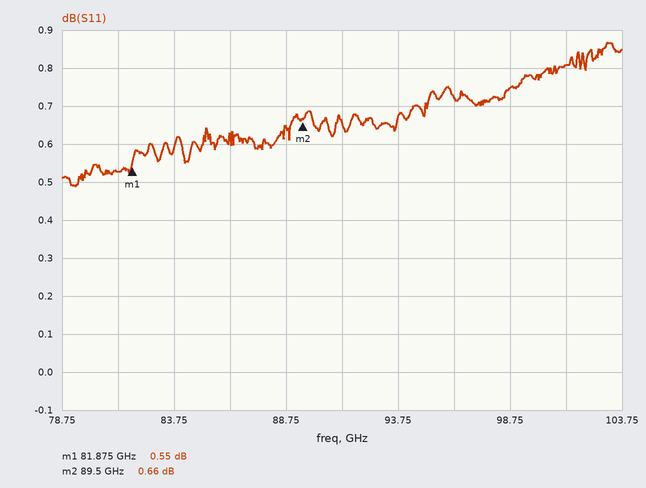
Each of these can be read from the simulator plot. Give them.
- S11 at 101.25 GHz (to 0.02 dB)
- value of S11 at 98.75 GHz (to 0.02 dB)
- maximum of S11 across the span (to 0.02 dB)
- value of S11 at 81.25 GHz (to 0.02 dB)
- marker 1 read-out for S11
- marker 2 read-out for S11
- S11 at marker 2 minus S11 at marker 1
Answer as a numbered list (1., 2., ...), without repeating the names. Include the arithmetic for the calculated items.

1. 0.80 dB
2. 0.74 dB
3. 0.86 dB
4. 0.52 dB
5. 0.55 dB
6. 0.66 dB
7. 0.66 − (0.55) = 0.11 dB
